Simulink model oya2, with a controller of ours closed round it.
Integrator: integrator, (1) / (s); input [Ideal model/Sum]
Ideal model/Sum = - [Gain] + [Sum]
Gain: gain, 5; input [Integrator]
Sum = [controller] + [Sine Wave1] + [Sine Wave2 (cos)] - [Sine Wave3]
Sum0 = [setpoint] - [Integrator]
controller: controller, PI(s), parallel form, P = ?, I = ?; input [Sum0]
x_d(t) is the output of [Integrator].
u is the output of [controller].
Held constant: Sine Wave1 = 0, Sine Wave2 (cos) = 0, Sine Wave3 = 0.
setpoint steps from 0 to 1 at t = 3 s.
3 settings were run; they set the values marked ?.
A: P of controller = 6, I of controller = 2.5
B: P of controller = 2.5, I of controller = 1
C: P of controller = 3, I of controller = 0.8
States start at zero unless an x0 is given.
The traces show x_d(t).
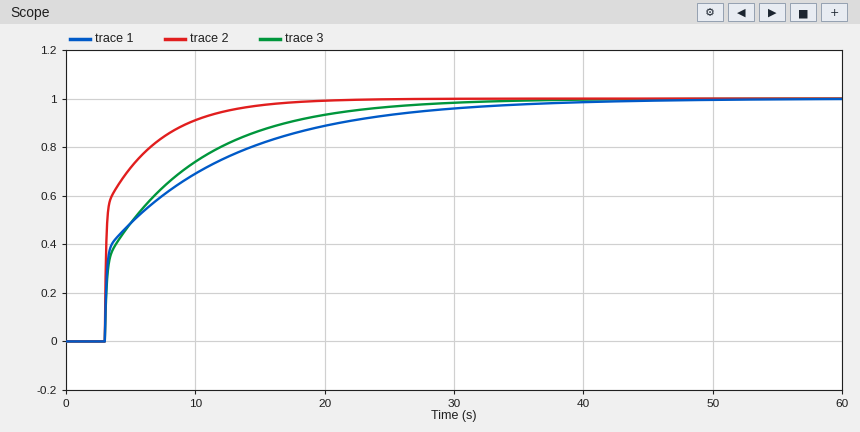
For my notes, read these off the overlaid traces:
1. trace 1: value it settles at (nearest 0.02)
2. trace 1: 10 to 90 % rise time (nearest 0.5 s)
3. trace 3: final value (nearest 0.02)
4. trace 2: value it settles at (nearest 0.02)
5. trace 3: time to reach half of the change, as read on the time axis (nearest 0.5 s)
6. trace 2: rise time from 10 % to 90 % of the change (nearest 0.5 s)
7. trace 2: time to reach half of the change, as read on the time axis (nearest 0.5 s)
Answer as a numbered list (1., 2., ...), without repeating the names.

1. 1.00
2. 18.0 s
3. 1.00
4. 1.00
5. 5.0 s
6. 6.5 s
7. 3.0 s
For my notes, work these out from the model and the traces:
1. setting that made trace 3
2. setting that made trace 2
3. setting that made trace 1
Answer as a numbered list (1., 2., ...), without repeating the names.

1. B
2. A
3. C
